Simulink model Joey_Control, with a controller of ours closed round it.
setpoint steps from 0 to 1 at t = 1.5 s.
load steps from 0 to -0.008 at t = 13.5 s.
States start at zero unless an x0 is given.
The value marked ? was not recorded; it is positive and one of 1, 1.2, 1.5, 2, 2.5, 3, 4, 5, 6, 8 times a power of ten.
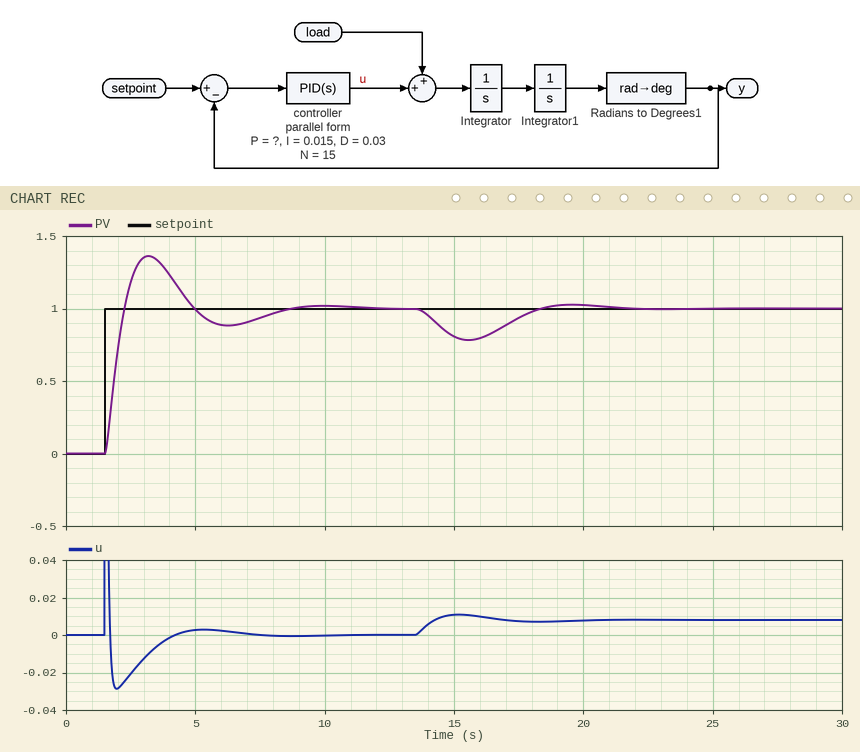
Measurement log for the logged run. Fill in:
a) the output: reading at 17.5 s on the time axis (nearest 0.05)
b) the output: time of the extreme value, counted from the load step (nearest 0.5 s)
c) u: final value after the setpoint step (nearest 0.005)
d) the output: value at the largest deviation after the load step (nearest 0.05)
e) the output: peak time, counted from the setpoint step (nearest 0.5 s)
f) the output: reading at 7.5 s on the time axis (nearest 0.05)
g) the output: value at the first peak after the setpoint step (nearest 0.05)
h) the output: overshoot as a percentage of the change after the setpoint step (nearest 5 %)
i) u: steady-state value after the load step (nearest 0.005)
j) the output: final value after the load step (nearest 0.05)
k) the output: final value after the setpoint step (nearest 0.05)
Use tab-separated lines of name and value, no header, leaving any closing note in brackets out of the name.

the output: reading at 17.5 s on the time axis	0.95
the output: time of the extreme value, counted from the load step	2.0 s
u: final value after the setpoint step	0.000
the output: value at the largest deviation after the load step	0.80
the output: peak time, counted from the setpoint step	1.5 s
the output: reading at 7.5 s on the time axis	0.95
the output: value at the first peak after the setpoint step	1.35
the output: overshoot as a percentage of the change after the setpoint step	35 %
u: steady-state value after the load step	0.010
the output: final value after the load step	1.00
the output: final value after the setpoint step	1.00
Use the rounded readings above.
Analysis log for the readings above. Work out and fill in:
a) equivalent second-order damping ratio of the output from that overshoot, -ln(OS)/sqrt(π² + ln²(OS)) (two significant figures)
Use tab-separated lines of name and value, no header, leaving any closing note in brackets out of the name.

equivalent second-order damping ratio of the output from that overshoot, -ln(OS)/sqrt(π² + ln²(OS))	0.32
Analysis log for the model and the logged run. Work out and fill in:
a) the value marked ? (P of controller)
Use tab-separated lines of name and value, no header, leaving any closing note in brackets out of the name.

the value marked ?	0.03
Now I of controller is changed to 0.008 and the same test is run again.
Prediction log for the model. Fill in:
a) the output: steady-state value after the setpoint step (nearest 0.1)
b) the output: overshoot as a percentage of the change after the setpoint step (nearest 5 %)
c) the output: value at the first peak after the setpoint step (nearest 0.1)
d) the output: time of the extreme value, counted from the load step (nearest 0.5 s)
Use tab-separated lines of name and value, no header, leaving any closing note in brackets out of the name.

the output: steady-state value after the setpoint step	1.0
the output: overshoot as a percentage of the change after the setpoint step	30 %
the output: value at the first peak after the setpoint step	1.3
the output: time of the extreme value, counted from the load step	2.5 s
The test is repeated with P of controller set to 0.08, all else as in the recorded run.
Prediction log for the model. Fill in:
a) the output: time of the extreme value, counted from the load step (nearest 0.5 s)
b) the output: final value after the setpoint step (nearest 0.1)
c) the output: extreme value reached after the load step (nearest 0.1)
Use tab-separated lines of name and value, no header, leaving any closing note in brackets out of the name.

the output: time of the extreme value, counted from the load step	1.5 s
the output: final value after the setpoint step	1.0
the output: extreme value reached after the load step	0.9
